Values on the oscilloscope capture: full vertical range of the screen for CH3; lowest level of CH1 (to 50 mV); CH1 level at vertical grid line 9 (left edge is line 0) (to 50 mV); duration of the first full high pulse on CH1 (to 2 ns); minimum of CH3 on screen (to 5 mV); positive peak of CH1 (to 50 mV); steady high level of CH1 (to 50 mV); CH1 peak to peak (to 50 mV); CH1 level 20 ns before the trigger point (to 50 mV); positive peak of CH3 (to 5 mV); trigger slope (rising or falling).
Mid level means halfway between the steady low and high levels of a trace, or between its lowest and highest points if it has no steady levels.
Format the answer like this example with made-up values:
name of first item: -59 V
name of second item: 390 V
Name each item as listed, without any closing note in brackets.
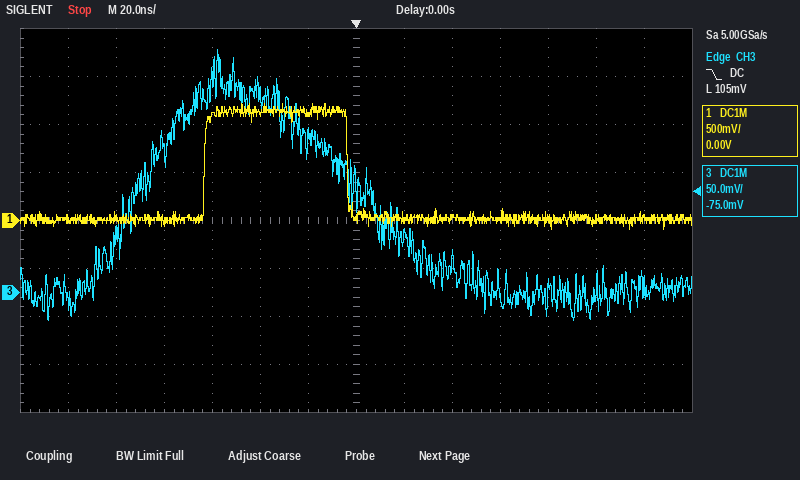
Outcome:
full vertical range of the screen for CH3: 400 mV
lowest level of CH1: -100 mV
CH1 level at vertical grid line 9 (left edge is line 0): 50 mV
duration of the first full high pulse on CH1: 60 ns
minimum of CH3 on screen: -30 mV
positive peak of CH1: 1.20 V
steady high level of CH1: 1.15 V
CH1 peak to peak: 1.30 V
CH1 level 20 ns before the trigger point: 1.10 V
positive peak of CH3: 255 mV
trigger slope: falling
